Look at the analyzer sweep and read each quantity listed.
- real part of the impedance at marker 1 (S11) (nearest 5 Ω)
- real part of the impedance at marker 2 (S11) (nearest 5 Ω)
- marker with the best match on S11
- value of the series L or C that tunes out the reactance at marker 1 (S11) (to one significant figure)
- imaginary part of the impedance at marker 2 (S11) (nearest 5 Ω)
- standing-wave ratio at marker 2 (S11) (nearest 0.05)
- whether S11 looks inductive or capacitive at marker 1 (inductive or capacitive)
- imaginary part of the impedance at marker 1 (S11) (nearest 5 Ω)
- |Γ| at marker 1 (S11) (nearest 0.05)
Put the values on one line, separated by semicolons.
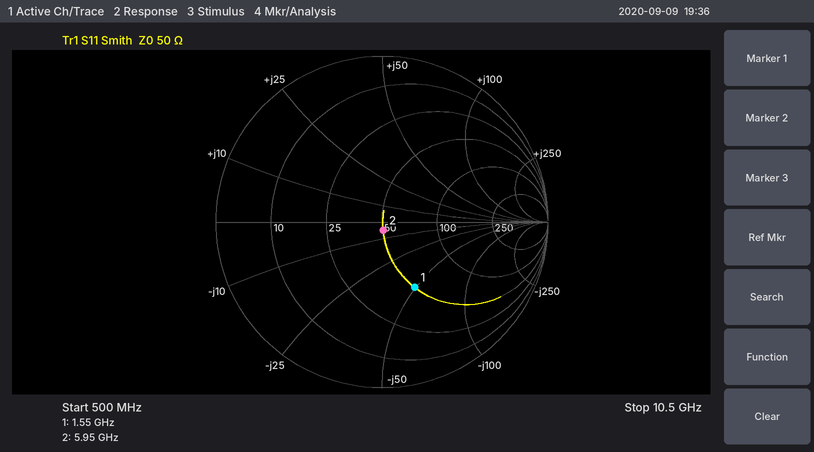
50 Ω; 50 Ω; marker 2; 5 nH; -5 Ω; 1.10; capacitive; -50 Ω; 0.45
